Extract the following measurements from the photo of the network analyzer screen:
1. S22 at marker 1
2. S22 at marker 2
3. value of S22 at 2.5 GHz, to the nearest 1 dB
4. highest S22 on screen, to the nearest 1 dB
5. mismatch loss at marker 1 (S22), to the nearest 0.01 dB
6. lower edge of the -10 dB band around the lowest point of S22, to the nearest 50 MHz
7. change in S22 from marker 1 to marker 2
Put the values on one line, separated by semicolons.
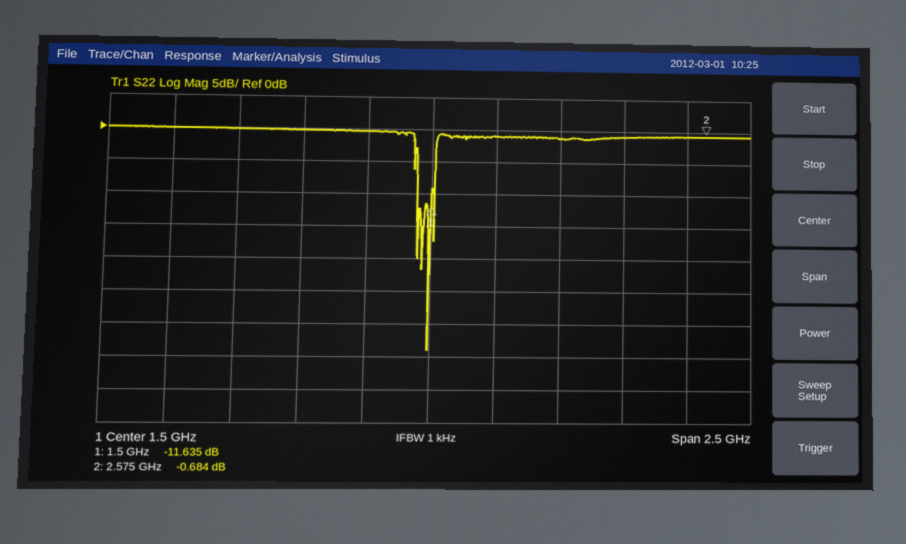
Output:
-11.635 dB; -0.684 dB; -1 dB; 0 dB; 0.31 dB; 1.45 GHz; 10.951 dB
